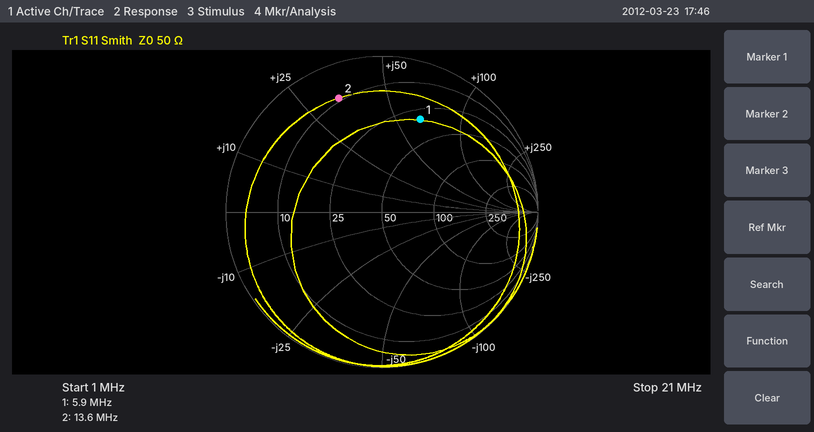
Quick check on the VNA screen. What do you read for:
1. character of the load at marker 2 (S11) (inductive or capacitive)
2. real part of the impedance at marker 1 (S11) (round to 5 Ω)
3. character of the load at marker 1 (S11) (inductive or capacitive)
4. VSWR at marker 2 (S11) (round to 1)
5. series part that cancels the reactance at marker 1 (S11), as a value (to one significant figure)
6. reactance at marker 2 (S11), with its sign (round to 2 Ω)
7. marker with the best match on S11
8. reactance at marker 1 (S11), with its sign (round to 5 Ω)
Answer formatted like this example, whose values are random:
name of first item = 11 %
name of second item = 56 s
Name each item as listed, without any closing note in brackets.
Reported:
character of the load at marker 2 (S11) = inductive
real part of the impedance at marker 1 (S11) = 30 Ω
character of the load at marker 1 (S11) = inductive
VSWR at marker 2 (S11) = 8
series part that cancels the reactance at marker 1 (S11), as a value = 400 pF
reactance at marker 2 (S11), with its sign = +34 Ω
marker with the best match on S11 = marker 1
reactance at marker 1 (S11), with its sign = +65 Ω
